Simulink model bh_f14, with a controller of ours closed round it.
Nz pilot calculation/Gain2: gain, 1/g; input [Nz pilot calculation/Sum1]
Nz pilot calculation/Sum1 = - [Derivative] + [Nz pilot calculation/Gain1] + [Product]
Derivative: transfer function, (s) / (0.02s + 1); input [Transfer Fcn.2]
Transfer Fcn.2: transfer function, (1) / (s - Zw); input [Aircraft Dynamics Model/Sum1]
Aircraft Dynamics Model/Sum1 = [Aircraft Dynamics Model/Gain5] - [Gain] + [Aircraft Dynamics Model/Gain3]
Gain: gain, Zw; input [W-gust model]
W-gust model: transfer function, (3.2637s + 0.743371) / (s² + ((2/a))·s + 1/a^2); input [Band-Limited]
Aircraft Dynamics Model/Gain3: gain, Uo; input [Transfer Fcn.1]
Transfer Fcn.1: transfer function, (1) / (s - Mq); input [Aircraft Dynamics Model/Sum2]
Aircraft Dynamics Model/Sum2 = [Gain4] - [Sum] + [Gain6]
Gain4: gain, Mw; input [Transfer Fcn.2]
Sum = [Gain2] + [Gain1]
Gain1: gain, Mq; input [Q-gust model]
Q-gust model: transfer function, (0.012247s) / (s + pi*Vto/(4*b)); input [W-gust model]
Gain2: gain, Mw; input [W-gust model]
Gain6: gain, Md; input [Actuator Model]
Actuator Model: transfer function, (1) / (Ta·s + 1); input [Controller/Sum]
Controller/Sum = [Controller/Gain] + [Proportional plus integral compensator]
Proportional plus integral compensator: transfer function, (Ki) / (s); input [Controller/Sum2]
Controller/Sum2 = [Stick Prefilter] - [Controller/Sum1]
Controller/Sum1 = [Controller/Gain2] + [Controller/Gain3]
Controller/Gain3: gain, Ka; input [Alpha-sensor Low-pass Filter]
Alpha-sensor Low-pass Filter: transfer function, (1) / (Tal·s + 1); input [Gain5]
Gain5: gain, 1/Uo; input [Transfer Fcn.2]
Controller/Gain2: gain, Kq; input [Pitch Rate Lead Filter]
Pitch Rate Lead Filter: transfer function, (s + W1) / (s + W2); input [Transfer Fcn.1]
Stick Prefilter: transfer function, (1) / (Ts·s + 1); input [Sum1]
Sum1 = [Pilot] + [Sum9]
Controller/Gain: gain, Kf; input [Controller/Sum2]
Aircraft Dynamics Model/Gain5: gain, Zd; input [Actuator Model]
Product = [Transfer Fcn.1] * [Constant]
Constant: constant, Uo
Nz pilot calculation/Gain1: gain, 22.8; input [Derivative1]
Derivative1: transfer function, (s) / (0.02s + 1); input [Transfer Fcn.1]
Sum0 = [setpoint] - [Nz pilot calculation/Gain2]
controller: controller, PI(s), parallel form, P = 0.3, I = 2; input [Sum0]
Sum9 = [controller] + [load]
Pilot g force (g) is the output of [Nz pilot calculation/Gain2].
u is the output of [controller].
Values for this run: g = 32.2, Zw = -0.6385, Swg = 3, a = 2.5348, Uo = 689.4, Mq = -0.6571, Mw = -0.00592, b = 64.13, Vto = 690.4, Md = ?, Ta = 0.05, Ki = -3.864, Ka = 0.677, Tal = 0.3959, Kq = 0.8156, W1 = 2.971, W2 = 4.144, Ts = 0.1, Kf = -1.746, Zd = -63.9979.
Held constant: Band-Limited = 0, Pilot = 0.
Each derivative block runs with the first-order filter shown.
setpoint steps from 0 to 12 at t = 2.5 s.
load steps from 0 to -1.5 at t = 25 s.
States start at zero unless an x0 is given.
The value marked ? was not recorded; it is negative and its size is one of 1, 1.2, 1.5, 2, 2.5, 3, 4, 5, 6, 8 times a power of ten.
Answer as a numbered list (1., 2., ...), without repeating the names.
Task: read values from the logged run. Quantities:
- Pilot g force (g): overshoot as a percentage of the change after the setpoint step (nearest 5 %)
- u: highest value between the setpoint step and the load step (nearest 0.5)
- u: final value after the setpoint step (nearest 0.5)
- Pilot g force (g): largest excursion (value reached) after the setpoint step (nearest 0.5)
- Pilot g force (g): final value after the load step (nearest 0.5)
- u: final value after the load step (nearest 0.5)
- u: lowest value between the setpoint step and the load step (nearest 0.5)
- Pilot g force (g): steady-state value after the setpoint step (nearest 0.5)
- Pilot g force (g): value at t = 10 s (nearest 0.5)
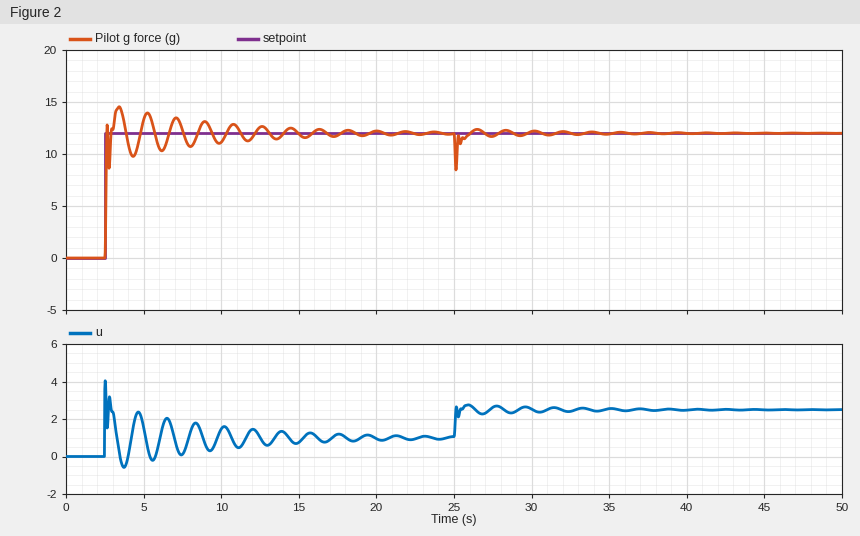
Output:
1. 20 %
2. 4.0
3. 1.0
4. 14.5
5. 12.0
6. 2.5
7. -0.5
8. 12.0
9. 11.0
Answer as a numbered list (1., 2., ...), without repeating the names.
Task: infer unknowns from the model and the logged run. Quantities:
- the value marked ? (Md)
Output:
1. -6
